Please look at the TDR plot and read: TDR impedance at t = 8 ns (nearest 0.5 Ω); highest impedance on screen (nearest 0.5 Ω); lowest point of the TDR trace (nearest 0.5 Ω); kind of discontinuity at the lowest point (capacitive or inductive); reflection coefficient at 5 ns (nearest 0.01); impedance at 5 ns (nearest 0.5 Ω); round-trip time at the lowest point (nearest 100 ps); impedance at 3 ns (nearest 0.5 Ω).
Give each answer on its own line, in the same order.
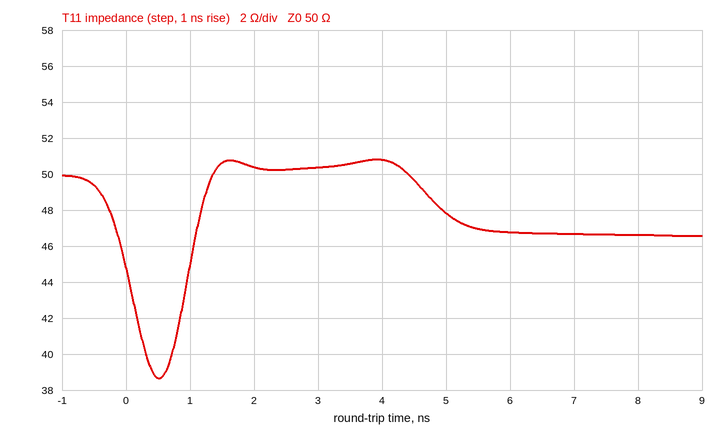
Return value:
46.5 Ω
51.0 Ω
38.5 Ω
capacitive
-0.02
48.0 Ω
500 ps
50.5 Ω
